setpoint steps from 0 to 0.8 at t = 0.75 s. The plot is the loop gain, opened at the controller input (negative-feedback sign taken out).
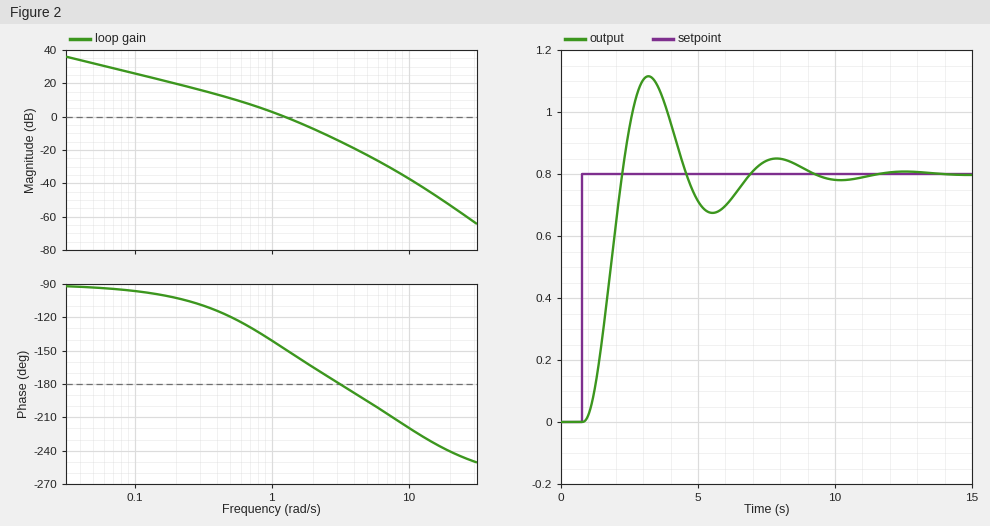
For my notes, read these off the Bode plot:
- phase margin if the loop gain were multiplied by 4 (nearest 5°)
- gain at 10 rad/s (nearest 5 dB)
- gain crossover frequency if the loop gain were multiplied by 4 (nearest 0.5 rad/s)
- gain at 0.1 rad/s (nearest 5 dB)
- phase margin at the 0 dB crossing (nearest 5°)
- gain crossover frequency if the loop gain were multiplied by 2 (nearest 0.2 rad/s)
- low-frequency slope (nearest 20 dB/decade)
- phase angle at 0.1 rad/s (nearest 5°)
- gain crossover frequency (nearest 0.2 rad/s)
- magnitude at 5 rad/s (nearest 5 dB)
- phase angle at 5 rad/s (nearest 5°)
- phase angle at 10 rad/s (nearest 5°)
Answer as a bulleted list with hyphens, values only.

- 5°
- -35 dB
- 2.5 rad/s
- 25 dB
- 30°
- 1.8 rad/s
- -20 dB/decade
- -95°
- 1.2 rad/s
- -25 dB
- -195°
- -220°
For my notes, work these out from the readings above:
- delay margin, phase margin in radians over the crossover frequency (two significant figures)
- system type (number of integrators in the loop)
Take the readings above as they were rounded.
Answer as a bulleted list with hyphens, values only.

- 0.44 s
- 1
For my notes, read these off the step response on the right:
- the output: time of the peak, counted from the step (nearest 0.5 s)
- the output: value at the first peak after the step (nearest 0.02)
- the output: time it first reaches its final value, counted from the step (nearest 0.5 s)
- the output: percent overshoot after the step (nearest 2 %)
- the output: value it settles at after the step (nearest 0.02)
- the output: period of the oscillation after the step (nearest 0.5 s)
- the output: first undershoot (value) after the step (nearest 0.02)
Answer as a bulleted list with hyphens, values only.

- 2.5 s
- 1.12
- 1.5 s
- 40 %
- 0.80
- 4.5 s
- 0.68
